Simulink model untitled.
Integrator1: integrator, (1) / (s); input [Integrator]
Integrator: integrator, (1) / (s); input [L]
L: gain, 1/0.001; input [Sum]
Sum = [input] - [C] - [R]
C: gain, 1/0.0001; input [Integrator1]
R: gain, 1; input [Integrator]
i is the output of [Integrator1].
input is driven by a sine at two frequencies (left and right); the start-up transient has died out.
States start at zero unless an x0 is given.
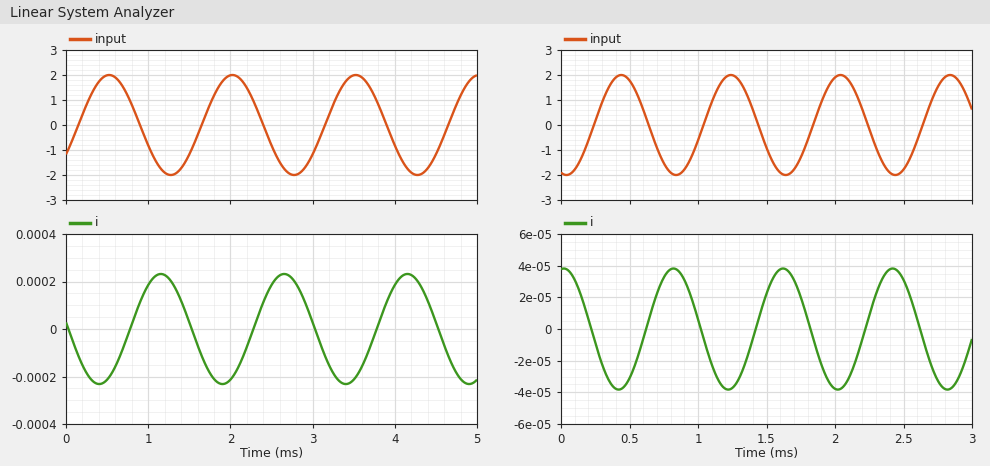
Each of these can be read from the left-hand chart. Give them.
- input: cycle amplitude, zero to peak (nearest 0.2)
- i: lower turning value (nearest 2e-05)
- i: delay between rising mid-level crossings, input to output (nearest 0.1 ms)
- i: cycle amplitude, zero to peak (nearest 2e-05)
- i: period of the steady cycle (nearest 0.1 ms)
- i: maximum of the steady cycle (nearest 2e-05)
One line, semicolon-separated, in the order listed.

2.0; -0.00024; 0.6 ms; 0.00024; 1.5 ms; 0.00024
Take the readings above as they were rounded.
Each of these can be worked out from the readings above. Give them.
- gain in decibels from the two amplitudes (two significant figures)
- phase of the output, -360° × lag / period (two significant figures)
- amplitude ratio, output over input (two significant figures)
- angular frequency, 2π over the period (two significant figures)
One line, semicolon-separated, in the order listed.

-78 dB; -140°; 0.00012; 4.2 rad/ms
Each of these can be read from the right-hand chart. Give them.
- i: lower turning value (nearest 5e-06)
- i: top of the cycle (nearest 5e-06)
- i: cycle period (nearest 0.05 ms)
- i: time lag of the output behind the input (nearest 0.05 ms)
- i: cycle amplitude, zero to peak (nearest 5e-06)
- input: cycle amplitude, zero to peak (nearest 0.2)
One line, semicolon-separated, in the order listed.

-0.000040; 0.000040; 0.80 ms; 0.40 ms; 0.000040; 2.0
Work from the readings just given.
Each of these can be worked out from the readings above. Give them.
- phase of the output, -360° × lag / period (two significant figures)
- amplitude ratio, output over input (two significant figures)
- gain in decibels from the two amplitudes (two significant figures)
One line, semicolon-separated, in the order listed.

-180°; 0.000020; -94 dB
